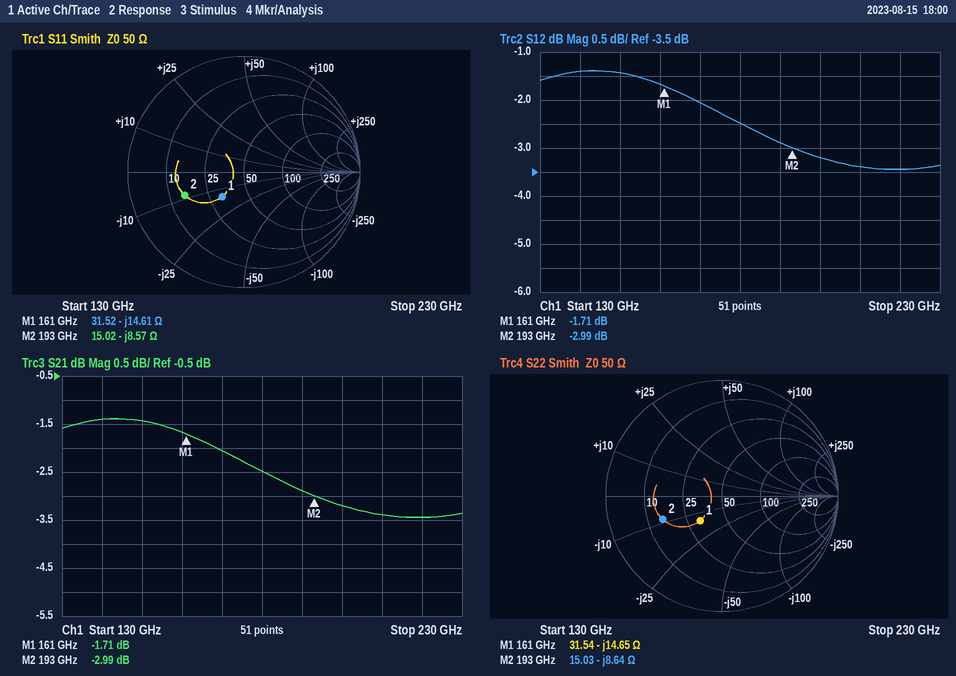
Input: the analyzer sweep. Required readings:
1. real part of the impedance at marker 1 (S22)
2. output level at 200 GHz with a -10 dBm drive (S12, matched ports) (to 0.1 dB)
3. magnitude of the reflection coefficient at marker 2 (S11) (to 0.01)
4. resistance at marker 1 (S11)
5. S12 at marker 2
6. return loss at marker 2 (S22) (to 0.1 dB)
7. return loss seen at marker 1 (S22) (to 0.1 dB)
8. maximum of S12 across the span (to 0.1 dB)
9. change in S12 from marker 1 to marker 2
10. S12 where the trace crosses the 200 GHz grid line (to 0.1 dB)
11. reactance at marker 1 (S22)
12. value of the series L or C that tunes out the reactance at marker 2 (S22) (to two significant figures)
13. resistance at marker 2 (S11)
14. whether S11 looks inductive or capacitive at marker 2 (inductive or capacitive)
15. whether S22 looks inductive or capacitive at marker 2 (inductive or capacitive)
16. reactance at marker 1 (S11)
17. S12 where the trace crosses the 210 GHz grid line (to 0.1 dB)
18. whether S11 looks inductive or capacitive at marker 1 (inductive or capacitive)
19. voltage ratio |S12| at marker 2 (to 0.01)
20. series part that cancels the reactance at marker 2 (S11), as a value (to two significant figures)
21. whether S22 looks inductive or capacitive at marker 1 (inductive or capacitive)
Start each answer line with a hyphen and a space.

- 31.54 Ω
- -13.2 dBm
- 0.55
- 31.52 Ω
- -2.99 dB
- 5.2 dB
- 10.9 dB
- -1.4 dB
- -1.28 dB
- -3.2 dB
- -14.65 Ω
- 7.1 pH
- 15.02 Ω
- capacitive
- capacitive
- -14.61 Ω
- -3.4 dB
- capacitive
- 0.71
- 7.1 pH
- capacitive
